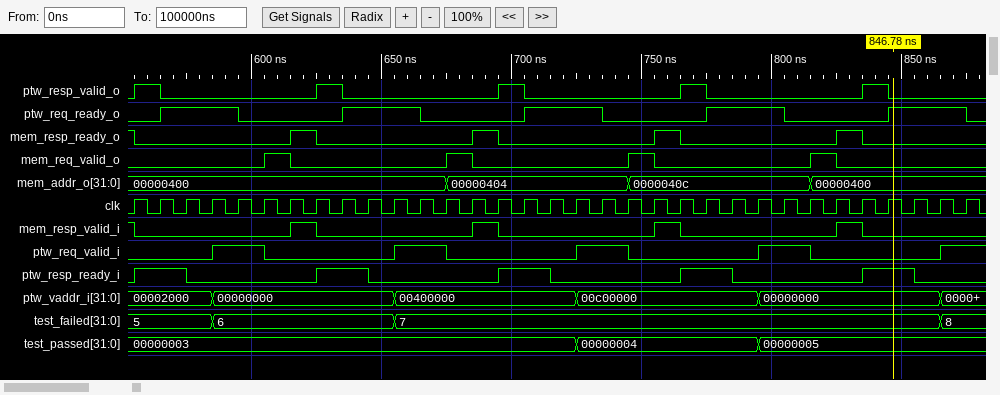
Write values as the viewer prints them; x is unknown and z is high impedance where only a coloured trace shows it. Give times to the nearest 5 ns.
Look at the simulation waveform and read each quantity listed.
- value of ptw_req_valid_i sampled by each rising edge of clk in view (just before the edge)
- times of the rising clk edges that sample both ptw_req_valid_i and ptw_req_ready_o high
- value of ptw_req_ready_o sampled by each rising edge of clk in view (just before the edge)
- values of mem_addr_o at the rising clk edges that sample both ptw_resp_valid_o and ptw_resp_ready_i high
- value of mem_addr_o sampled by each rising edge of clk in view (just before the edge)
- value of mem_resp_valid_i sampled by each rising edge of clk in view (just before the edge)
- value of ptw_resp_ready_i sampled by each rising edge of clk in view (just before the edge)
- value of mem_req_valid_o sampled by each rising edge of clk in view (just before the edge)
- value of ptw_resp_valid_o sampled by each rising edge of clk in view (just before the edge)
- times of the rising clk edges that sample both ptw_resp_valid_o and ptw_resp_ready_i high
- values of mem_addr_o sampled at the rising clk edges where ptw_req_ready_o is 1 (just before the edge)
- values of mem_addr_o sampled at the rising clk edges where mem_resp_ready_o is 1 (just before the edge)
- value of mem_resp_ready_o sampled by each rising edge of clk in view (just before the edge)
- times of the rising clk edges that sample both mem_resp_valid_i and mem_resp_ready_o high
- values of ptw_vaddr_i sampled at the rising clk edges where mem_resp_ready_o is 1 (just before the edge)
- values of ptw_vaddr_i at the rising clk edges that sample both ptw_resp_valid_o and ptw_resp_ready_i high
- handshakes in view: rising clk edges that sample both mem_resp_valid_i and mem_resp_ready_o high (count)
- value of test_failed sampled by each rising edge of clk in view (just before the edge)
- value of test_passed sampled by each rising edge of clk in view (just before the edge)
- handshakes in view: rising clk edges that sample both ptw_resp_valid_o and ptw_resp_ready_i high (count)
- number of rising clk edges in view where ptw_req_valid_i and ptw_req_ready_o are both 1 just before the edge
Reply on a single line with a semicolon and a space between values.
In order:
0 0 0 0 1 1 0 0 0 0 0 1 1 0 0 0 0 0 1 1 0 0 0 0 0 1 1 0 0 0 0 0 1; 595 ns, 665 ns, 735 ns, 805 ns, 875 ns; 0 0 1 1 1 0 0 0 0 1 1 1 0 0 0 0 1 1 1 0 0 0 0 1 1 1 0 0 0 0 1 1 1; 00000400, 00000400, 00000404, 0000040c, 00000400; 00000400, 00000400, 00000400, 00000400, 00000400, 00000400, 00000400, 00000400, 00000400, 00000400, 00000400, 00000400, 00000400, 00000404, 00000404, 00000404, 00000404, 00000404, 00000404, 00000404, 0000040c, 0000040c, 0000040c, 0000040c, 0000040c, 0000040c, 0000040c, 00000400, 00000400, 00000400, 00000400, 00000400, 00000400; 1 0 0 0 0 0 0 1 0 0 0 0 0 0 1 0 0 0 0 0 0 1 0 0 0 0 0 0 1 0 0 0 0; 0 1 1 0 0 0 0 0 1 1 0 0 0 0 0 1 1 0 0 0 0 0 1 1 0 0 0 0 0 1 1 0 0; 0 0 0 0 0 0 1 0 0 0 0 0 0 1 0 0 0 0 0 0 1 0 0 0 0 0 0 1 0 0 0 0 0; 0 1 0 0 0 0 0 0 1 0 0 0 0 0 0 1 0 0 0 0 0 0 1 0 0 0 0 0 0 1 0 0 0; 565 ns, 635 ns, 705 ns, 775 ns, 845 ns; 00000400, 00000400, 00000400, 00000400, 00000400, 00000400, 00000404, 00000404, 00000404, 0000040c, 0000040c, 0000040c, 00000400, 00000400, 00000400; 00000400, 00000400, 00000404, 0000040c, 00000400; 1 0 0 0 0 0 0 1 0 0 0 0 0 0 1 0 0 0 0 0 0 1 0 0 0 0 0 0 1 0 0 0 0; 555 ns, 625 ns, 695 ns, 765 ns, 835 ns; 00002000, 00000000, 00400000, 00c00000, 00000000; 00002000, 00000000, 00400000, 00c00000, 00000000; 5; 5, 5, 5, 5, 6, 6, 6, 6, 6, 6, 6, 7, 7, 7, 7, 7, 7, 7, 7, 7, 7, 7, 7, 7, 7, 7, 7, 7, 7, 7, 7, 7, 8; 00000003, 00000003, 00000003, 00000003, 00000003, 00000003, 00000003, 00000003, 00000003, 00000003, 00000003, 00000003, 00000003, 00000003, 00000003, 00000003, 00000003, 00000003, 00000004, 00000004, 00000004, 00000004, 00000004, 00000004, 00000004, 00000005, 00000005, 00000005, 00000005, 00000005, 00000005, 00000005, 00000005; 5; 5
